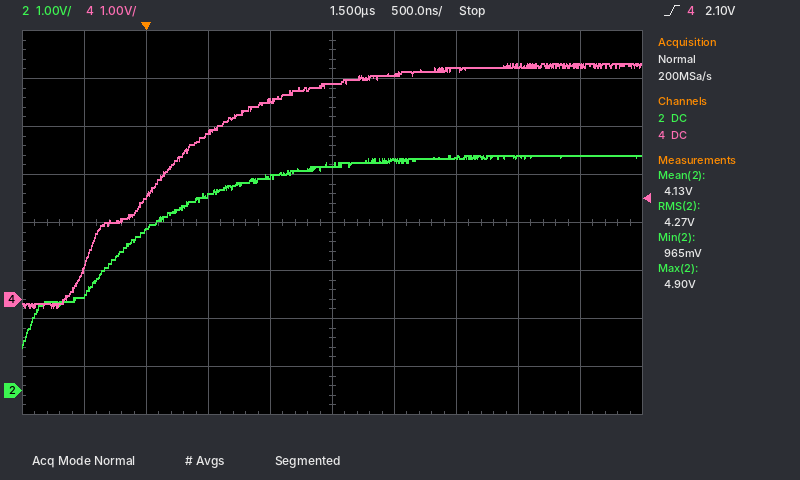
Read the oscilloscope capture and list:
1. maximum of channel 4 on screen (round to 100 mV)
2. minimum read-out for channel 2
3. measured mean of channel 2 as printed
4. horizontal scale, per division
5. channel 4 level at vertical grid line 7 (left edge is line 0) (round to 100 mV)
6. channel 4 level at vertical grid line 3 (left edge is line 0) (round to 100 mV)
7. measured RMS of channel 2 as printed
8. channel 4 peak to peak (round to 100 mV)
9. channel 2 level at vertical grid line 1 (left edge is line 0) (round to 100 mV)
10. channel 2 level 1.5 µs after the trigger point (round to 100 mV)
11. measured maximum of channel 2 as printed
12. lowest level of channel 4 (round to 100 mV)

4.9 V
965 mV
4.13 V
500 ns
4.8 V
3.5 V
4.27 V
5.1 V
2.0 V
4.7 V
4.90 V
-200 mV
